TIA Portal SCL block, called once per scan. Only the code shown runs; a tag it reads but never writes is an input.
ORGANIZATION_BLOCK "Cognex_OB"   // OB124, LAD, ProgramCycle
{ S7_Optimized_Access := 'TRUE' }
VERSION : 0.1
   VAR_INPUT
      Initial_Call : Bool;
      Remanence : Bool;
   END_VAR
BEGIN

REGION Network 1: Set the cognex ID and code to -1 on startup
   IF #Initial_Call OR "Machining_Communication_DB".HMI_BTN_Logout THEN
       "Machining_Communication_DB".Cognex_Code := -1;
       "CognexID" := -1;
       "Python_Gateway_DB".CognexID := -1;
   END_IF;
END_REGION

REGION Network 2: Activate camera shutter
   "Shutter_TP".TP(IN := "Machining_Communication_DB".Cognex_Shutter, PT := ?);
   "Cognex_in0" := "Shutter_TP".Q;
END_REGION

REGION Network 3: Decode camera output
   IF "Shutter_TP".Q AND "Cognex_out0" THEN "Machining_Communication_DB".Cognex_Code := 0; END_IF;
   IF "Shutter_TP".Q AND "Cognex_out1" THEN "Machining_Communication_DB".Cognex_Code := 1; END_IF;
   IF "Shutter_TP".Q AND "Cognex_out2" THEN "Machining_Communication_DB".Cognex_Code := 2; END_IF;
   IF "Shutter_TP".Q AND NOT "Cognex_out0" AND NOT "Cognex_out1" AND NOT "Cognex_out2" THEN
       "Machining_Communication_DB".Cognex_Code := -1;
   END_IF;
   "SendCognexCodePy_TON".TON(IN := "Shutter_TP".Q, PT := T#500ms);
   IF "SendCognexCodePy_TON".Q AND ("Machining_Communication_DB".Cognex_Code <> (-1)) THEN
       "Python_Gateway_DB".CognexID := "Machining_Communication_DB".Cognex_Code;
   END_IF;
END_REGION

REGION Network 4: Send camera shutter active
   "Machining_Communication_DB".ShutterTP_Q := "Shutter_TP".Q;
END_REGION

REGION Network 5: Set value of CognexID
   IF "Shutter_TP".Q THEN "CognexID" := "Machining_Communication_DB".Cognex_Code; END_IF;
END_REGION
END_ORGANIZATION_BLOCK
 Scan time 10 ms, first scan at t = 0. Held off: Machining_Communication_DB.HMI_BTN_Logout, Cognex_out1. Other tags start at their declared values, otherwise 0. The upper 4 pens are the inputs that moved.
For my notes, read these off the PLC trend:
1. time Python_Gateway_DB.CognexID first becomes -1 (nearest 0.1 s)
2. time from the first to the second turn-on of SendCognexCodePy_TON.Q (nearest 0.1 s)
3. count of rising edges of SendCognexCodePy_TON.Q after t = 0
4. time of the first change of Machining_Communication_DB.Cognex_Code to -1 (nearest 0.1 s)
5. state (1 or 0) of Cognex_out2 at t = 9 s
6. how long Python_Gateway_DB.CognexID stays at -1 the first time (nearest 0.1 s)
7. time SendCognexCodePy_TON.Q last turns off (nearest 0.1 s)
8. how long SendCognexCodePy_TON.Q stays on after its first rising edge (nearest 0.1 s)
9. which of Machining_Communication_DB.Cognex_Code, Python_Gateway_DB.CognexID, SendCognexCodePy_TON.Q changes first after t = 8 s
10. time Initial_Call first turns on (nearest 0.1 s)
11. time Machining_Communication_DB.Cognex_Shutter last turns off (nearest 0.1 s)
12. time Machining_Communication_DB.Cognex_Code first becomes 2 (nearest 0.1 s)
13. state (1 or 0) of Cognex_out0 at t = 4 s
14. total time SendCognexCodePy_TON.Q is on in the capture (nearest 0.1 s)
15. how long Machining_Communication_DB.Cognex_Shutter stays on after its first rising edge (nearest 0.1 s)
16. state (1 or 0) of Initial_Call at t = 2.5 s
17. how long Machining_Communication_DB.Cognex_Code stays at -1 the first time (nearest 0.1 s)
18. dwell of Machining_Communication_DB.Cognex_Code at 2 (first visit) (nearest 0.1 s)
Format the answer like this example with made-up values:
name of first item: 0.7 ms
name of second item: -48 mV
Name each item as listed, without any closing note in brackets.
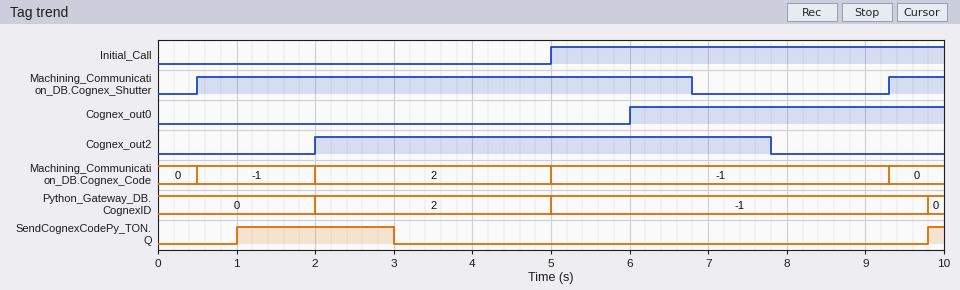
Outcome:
time Python_Gateway_DB.CognexID first becomes -1: 5.0 s
time from the first to the second turn-on of SendCognexCodePy_TON.Q: 8.8 s
count of rising edges of SendCognexCodePy_TON.Q after t = 0: 2
time of the first change of Machining_Communication_DB.Cognex_Code to -1: 0.5 s
state (1 or 0) of Cognex_out2 at t = 9 s: 0
how long Python_Gateway_DB.CognexID stays at -1 the first time: 4.8 s
time SendCognexCodePy_TON.Q last turns off: 3.0 s
how long SendCognexCodePy_TON.Q stays on after its first rising edge: 2.0 s
which of Machining_Communication_DB.Cognex_Code, Python_Gateway_DB.CognexID, SendCognexCodePy_TON.Q changes first after t = 8 s: Machining_Communication_DB.Cognex_Code
time Initial_Call first turns on: 5.0 s
time Machining_Communication_DB.Cognex_Shutter last turns off: 6.8 s
time Machining_Communication_DB.Cognex_Code first becomes 2: 2.0 s
state (1 or 0) of Cognex_out0 at t = 4 s: 0
total time SendCognexCodePy_TON.Q is on in the capture: 2.2 s
how long Machining_Communication_DB.Cognex_Shutter stays on after its first rising edge: 6.3 s
state (1 or 0) of Initial_Call at t = 2.5 s: 0
how long Machining_Communication_DB.Cognex_Code stays at -1 the first time: 1.5 s
dwell of Machining_Communication_DB.Cognex_Code at 2 (first visit): 3.0 s
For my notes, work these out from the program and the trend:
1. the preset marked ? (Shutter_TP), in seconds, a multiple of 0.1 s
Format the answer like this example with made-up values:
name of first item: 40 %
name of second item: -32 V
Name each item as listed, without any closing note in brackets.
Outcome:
the preset marked ? (Shutter_TP), in seconds, a multiple of 0.1 s: 2.5 s
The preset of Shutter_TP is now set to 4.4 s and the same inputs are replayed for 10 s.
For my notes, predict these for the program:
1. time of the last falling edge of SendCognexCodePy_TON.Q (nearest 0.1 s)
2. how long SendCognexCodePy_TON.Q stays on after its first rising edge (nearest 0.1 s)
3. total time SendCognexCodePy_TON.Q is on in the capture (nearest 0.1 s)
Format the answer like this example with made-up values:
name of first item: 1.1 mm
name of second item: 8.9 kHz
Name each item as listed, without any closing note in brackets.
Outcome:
time of the last falling edge of SendCognexCodePy_TON.Q: 4.9 s
how long SendCognexCodePy_TON.Q stays on after its first rising edge: 3.9 s
total time SendCognexCodePy_TON.Q is on in the capture: 4.1 s
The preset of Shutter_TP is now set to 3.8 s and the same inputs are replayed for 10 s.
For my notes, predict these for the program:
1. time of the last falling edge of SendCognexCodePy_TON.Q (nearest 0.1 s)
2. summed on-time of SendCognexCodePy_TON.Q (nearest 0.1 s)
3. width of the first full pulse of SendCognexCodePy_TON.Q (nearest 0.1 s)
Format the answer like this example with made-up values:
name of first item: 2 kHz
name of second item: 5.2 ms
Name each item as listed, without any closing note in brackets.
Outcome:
time of the last falling edge of SendCognexCodePy_TON.Q: 4.3 s
summed on-time of SendCognexCodePy_TON.Q: 3.5 s
width of the first full pulse of SendCognexCodePy_TON.Q: 3.3 s
